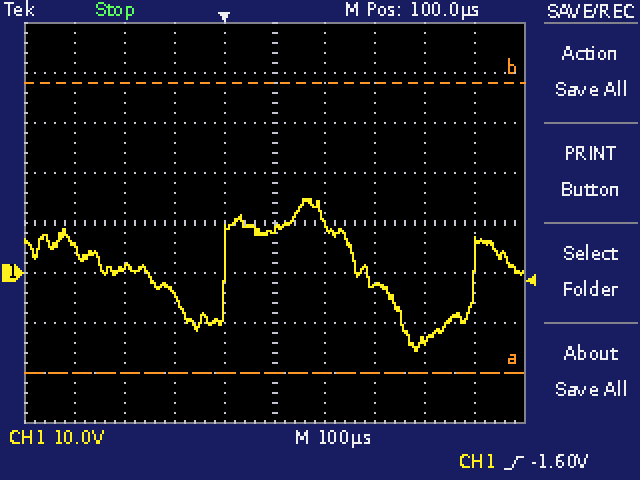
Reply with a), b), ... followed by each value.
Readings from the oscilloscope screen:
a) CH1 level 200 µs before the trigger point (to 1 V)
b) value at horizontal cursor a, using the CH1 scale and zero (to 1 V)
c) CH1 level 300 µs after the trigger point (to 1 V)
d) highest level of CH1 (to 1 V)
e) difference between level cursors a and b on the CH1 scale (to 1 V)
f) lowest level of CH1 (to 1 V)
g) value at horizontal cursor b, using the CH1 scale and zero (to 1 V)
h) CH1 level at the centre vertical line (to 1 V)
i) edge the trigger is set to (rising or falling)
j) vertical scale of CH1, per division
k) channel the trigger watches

a) 1 V
b) -20 V
c) -2 V
d) 15 V
e) 58 V
f) -16 V
g) 38 V
h) 9 V
i) rising
j) 10 V
k) CH1
